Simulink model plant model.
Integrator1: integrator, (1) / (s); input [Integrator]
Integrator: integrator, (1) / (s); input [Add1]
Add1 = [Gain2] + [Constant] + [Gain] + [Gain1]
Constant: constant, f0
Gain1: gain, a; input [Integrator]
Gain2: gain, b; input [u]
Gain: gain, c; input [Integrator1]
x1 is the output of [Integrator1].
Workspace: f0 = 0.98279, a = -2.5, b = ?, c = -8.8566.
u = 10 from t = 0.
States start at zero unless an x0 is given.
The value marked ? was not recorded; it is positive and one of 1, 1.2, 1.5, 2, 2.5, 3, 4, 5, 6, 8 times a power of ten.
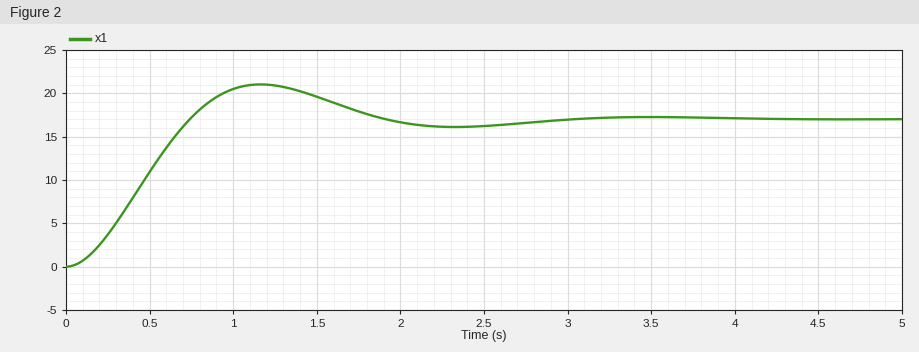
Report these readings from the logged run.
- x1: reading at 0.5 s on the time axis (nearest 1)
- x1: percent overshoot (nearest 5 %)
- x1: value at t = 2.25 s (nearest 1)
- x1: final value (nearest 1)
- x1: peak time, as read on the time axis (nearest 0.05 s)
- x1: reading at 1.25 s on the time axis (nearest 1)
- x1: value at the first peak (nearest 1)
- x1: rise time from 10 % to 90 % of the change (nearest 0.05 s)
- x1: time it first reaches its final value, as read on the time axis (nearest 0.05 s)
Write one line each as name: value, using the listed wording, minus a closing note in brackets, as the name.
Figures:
x1: reading at 0.5 s on the time axis: 11
x1: percent overshoot: 25 %
x1: value at t = 2.25 s: 16
x1: final value: 17
x1: peak time, as read on the time axis: 1.15 s
x1: reading at 1.25 s on the time axis: 21
x1: value at the first peak: 21
x1: rise time from 10 % to 90 % of the change: 0.50 s
x1: time it first reaches its final value, as read on the time axis: 0.75 s
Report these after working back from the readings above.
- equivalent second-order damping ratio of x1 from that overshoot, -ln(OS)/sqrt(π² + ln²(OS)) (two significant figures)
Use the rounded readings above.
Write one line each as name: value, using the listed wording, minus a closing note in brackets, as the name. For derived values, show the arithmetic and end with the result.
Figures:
equivalent second-order damping ratio of x1 from that overshoot, -ln(OS)/sqrt(π² + ln²(OS)): ln(0.25) = -1.386; 1.386 / sqrt(9.870 + 1.922) = 0.40
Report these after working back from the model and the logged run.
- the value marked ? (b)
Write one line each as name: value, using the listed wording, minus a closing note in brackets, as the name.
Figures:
the value marked ?: 15
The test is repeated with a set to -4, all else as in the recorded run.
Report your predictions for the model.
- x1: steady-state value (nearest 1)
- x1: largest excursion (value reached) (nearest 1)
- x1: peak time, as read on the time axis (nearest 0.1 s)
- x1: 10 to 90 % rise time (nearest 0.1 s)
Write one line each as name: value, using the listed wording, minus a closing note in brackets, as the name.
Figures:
x1: steady-state value: 17
x1: largest excursion (value reached): 18
x1: peak time, as read on the time axis: 1.4 s
x1: 10 to 90 % rise time: 0.7 s
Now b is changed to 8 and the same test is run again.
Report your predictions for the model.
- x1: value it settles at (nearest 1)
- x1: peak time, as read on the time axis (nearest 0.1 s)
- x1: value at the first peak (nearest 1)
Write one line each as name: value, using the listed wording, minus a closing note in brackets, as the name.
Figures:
x1: value it settles at: 9
x1: peak time, as read on the time axis: 1.2 s
x1: value at the first peak: 11
